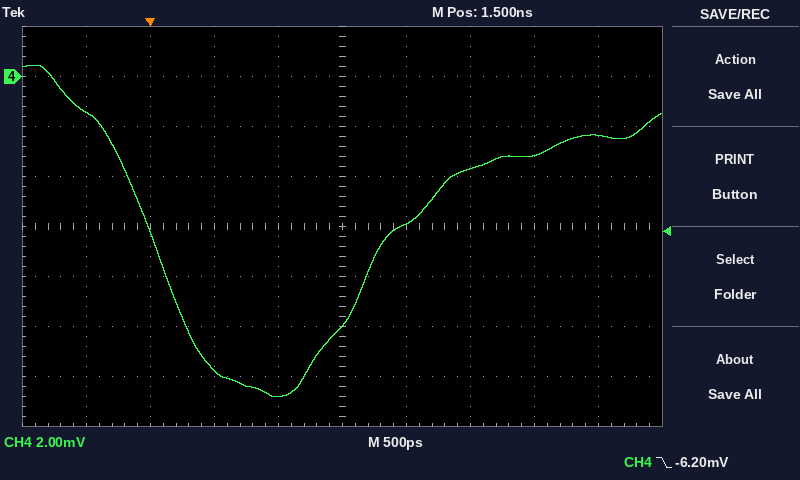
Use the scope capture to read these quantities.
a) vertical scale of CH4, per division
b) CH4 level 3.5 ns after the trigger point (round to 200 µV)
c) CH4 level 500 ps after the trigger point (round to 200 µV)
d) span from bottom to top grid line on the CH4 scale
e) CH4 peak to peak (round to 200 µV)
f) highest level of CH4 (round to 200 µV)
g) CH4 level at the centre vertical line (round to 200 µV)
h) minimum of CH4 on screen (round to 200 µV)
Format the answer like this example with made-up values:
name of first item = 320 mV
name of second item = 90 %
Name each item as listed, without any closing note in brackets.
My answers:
vertical scale of CH4, per division = 2 mV
CH4 level 3.5 ns after the trigger point = -2.4 mV
CH4 level 500 ps after the trigger point = -11.8 mV
span from bottom to top grid line on the CH4 scale = 16 mV
CH4 peak to peak = 13.2 mV
highest level of CH4 = 400 µV
CH4 level at the centre vertical line = -10.0 mV
minimum of CH4 on screen = -12.8 mV
